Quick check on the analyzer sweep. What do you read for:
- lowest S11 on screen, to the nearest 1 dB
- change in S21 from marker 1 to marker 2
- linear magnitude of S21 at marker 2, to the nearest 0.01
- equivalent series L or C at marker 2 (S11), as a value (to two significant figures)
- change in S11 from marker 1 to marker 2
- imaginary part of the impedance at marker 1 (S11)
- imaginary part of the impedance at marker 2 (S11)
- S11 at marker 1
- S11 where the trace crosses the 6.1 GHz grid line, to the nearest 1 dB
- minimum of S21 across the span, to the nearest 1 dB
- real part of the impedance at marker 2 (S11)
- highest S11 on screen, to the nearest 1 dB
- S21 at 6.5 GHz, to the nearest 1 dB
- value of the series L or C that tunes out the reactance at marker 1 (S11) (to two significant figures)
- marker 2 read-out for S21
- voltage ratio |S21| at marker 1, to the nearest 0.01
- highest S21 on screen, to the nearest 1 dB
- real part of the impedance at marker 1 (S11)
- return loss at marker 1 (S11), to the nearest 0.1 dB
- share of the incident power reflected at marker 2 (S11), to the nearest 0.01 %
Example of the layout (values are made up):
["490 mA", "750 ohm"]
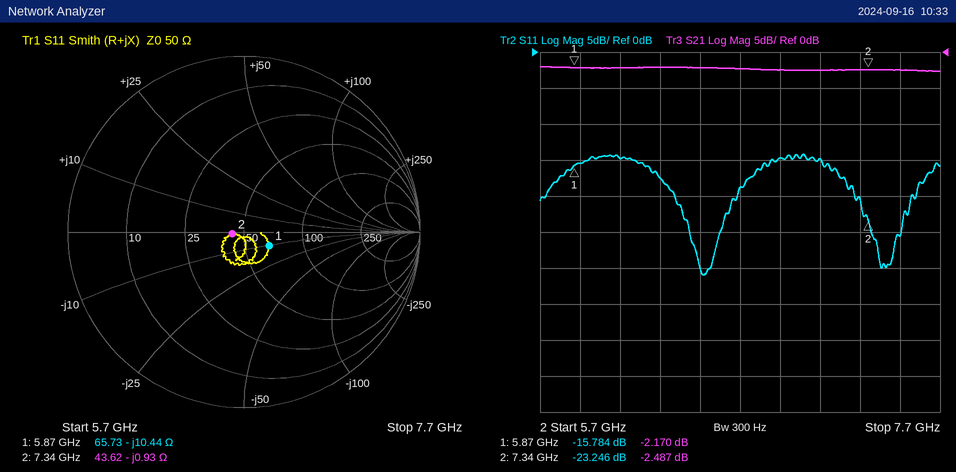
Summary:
["-31 dB", "-0.317 dB", "0.75", "23 pF", "-7.462 dB", "-10.44 Ω", "-0.93 Ω", "-15.784 dB", "-15 dB", "-3 dB", "43.62 Ω", "-14 dB", "-2 dB", "280 pH", "-2.487 dB", "0.78", "-2 dB", "65.73 Ω", "15.8 dB", "0.47 %"]
